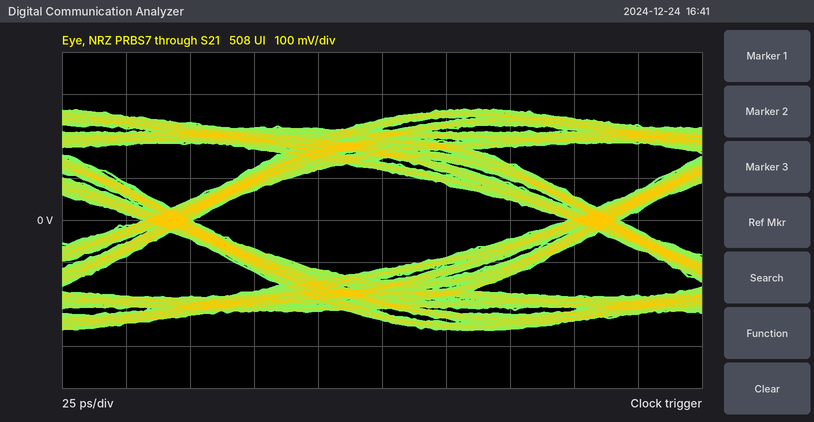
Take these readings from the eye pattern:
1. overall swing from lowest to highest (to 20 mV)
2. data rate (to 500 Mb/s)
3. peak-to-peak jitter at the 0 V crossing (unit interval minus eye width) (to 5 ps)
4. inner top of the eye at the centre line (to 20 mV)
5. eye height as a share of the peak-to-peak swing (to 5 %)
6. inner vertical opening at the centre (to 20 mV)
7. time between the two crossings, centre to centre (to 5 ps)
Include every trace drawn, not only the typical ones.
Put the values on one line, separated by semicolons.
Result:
520 mV; 6.0 Gb/s; 20 ps; 120 mV; 45 %; 240 mV; 165 ps
